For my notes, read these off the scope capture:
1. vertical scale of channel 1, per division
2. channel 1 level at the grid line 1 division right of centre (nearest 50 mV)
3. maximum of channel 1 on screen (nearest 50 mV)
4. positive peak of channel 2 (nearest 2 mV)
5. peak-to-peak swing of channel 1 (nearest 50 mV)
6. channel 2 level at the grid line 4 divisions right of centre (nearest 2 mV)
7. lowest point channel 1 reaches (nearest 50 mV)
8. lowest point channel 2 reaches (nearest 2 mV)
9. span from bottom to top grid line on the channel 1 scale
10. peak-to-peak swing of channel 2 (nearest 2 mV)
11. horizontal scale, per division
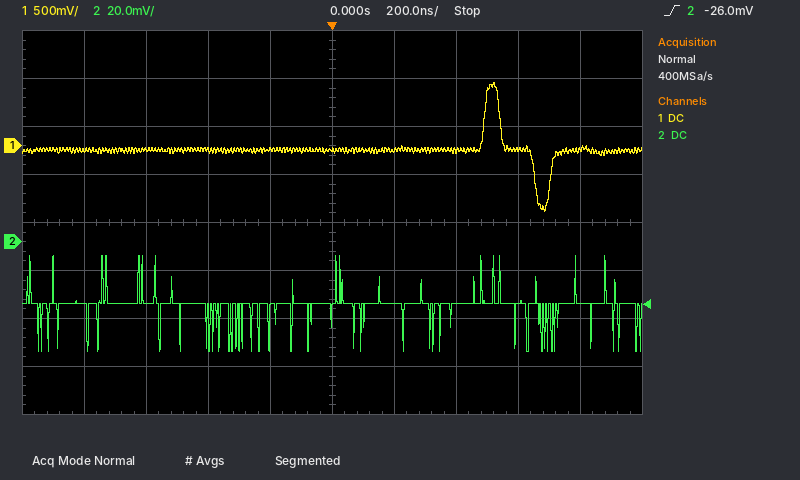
500 mV
-50 mV
650 mV
-6 mV
1.35 V
-26 mV
-700 mV
-46 mV
4 V
40 mV
200 ns
